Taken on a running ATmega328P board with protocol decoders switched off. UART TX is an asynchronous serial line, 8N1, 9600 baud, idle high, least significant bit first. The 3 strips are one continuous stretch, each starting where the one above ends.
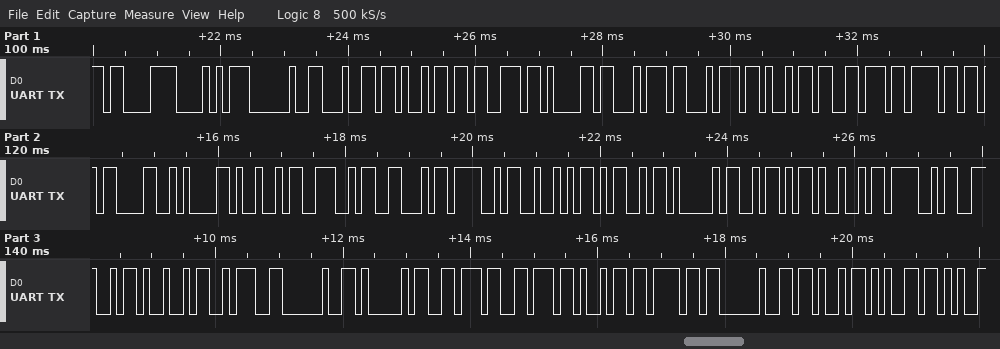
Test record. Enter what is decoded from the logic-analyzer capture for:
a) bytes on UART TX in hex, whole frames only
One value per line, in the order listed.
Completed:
C3 A8 20 64 69 73 61 74 74 69 76 6F 0D 0A 49 4E 46 4F 52 4D 41 5A 49 4F 4E 49 3A 20 41 76 76 69 6F 20 4B 65
